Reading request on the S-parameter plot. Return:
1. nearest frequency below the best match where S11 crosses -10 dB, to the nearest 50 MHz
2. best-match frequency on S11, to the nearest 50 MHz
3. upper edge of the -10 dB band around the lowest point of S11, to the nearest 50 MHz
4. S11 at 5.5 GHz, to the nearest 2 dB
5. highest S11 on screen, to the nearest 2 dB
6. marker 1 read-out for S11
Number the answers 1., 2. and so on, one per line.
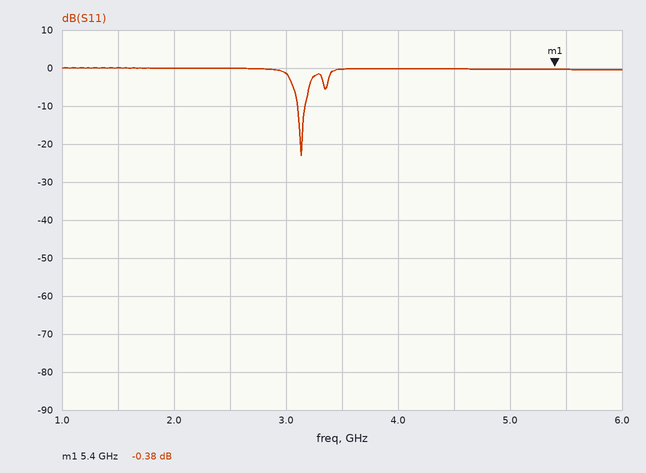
1. 3.10 GHz
2. 3.15 GHz
3. 3.15 GHz
4. 0 dB
5. 0 dB
6. -0.38 dB
